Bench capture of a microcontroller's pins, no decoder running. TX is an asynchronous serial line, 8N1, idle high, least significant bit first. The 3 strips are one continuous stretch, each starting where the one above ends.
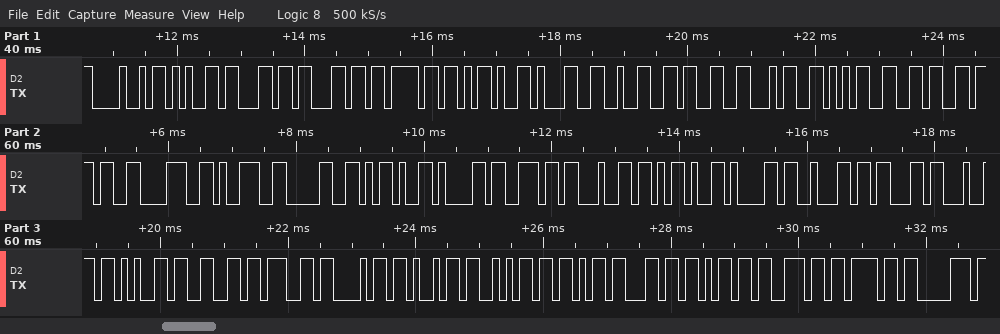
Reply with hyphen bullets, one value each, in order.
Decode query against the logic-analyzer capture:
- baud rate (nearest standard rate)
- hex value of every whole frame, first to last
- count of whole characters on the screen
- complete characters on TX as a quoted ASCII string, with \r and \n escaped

- 9600 baud
- 48 65 6C 6C 6F 2D 31 32 33 34 35 36 37 38 39 30 2D 61 6E 64 2D 61 62 63 64 65 66 67 68 69 6A 6B 6C 6D 6E 6F 70
- 37
- "Hello-1234567890-and-abcdefghijklmnop"
